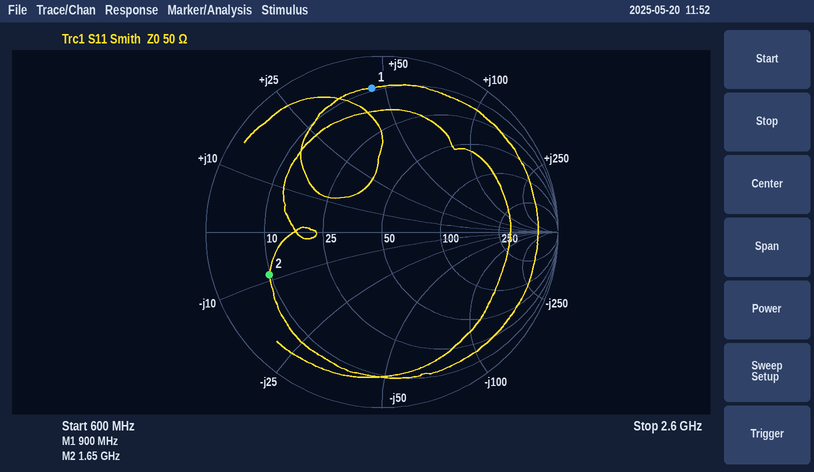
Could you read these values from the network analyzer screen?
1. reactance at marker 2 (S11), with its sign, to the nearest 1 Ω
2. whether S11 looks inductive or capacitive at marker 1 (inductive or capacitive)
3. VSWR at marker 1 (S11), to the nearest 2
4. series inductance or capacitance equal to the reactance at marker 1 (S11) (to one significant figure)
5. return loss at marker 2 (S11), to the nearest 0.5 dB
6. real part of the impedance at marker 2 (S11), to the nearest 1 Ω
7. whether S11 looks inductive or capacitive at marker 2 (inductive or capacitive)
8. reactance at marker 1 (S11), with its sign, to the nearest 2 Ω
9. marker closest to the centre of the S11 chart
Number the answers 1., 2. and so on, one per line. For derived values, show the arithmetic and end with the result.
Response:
1. -9 Ω
2. inductive
3. 10
4. L = 46 Ω/(2π × 900 MHz) ≈ 8 nH
5. 3.5 dB
6. 10 Ω
7. capacitive
8. +46 Ω
9. marker 2
